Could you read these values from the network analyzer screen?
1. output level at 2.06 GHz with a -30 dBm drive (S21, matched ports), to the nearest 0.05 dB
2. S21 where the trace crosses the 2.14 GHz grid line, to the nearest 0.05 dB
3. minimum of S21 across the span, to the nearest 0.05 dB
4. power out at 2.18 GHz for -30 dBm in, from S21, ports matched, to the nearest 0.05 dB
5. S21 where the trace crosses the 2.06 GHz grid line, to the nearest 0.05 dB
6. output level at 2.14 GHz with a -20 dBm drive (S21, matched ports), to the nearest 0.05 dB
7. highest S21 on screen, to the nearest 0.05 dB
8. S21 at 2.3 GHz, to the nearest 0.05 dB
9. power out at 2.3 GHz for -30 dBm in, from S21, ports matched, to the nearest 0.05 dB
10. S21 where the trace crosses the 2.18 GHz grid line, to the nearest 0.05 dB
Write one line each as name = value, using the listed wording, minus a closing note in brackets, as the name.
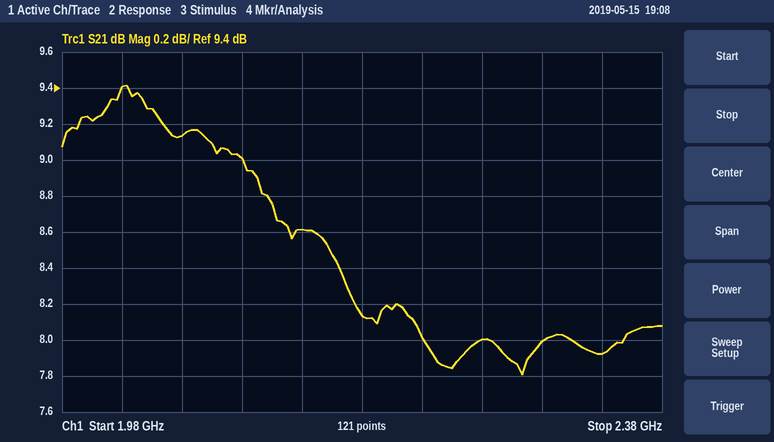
output level at 2.06 GHz with a -30 dBm drive (S21, matched ports), to the nearest 0.05 dB = -20.85 dBm
S21 where the trace crosses the 2.14 GHz grid line, to the nearest 0.05 dB = 8.60 dB
minimum of S21 across the span, to the nearest 0.05 dB = 7.80 dB
power out at 2.18 GHz for -30 dBm in, from S21, ports matched, to the nearest 0.05 dB = -21.85 dBm
S21 where the trace crosses the 2.06 GHz grid line, to the nearest 0.05 dB = 9.15 dB
output level at 2.14 GHz with a -20 dBm drive (S21, matched ports), to the nearest 0.05 dB = -11.40 dBm
highest S21 on screen, to the nearest 0.05 dB = 9.40 dB
S21 at 2.3 GHz, to the nearest 0.05 dB = 8.00 dB
power out at 2.3 GHz for -30 dBm in, from S21, ports matched, to the nearest 0.05 dB = -22.00 dBm
S21 where the trace crosses the 2.18 GHz grid line, to the nearest 0.05 dB = 8.15 dB
